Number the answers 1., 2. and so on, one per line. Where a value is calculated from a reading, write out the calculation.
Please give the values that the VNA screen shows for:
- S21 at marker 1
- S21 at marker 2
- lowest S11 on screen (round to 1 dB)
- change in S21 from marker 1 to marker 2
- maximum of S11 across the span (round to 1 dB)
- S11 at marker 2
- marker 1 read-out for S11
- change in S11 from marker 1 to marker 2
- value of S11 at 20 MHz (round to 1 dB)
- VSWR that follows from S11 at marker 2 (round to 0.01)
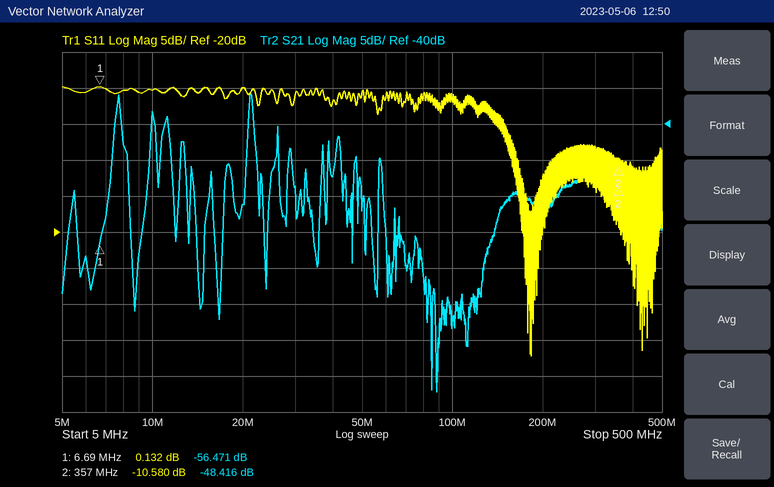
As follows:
1. -56.471 dB
2. -48.416 dB
3. -37 dB
4. -48.416 − (-56.471) = 8.055 dB
5. 0 dB
6. -10.580 dB
7. 0.132 dB
8. -10.58 − (0.132) = -10.712 dB
9. 0 dB
10. (1 + 0.2958)/(1 − 0.2958) ≈ 1.84
